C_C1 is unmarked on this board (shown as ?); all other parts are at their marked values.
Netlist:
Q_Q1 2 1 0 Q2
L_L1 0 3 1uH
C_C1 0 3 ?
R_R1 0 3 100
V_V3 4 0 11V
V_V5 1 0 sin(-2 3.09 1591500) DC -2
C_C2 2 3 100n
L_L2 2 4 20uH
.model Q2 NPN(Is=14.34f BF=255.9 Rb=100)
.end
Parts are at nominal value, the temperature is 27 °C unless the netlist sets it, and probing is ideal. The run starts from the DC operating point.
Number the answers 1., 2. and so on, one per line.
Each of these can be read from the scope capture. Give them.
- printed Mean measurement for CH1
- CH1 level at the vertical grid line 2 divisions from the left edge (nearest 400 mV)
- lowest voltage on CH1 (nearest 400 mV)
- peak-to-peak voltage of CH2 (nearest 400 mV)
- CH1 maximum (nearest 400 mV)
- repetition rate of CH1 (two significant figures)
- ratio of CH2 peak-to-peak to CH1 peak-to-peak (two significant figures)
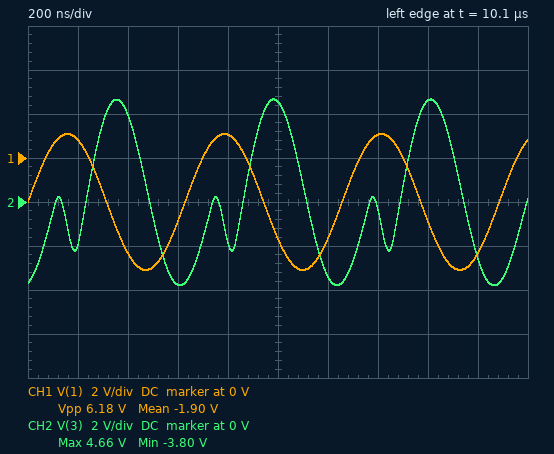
1. -1.90 V
2. -4.4 V
3. -5.2 V
4. 8.4 V
5. 1.2 V
6. 1.6 MHz
7. 1.4
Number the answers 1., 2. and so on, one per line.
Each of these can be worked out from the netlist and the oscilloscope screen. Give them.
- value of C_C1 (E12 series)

1. 6.8 nF
